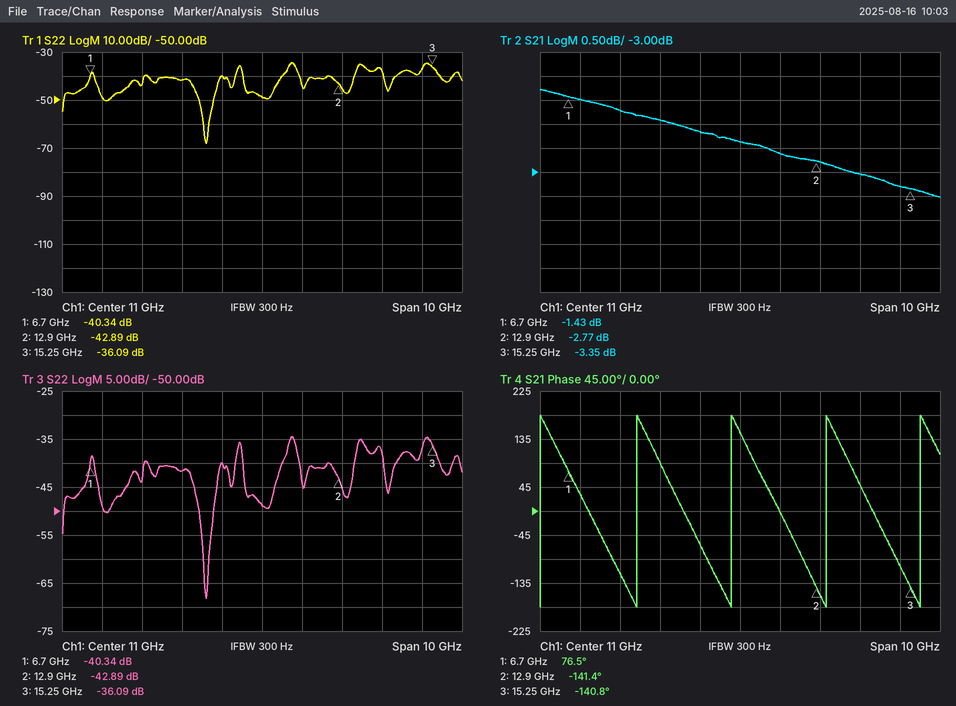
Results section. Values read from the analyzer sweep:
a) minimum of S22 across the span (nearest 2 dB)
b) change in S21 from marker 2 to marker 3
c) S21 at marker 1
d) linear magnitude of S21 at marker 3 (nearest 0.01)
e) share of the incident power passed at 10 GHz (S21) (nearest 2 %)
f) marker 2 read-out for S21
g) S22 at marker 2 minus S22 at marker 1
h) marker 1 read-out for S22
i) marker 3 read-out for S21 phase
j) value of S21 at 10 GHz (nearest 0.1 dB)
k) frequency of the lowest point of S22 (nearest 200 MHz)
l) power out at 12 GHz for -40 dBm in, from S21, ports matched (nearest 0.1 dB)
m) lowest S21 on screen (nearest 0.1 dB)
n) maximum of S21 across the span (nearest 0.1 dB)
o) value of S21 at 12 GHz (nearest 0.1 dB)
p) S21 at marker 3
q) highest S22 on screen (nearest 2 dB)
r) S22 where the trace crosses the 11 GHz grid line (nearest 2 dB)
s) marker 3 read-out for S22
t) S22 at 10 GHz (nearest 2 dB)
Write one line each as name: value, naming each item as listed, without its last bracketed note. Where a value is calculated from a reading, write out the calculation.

minimum of S22 across the span: -68 dB
change in S21 from marker 2 to marker 3: -3.35 − (-2.77) = -0.58 dB
S21 at marker 1: -1.43 dB
linear magnitude of S21 at marker 3: 10^(-3.35/20) ≈ 0.68
share of the incident power passed at 10 GHz (S21): 10^(-2.2/10) ≈ 60 %
marker 2 read-out for S21: -2.77 dB
S22 at marker 2 minus S22 at marker 1: -42.89 − (-40.34) = -2.55 dB
marker 1 read-out for S22: -40.34 dB
marker 3 read-out for S21 phase: -140.8°
value of S21 at 10 GHz: -2.2 dB
frequency of the lowest point of S22: 9.6 GHz
power out at 12 GHz for -40 dBm in, from S21, ports matched: -40 dBm + (-2.6 dB) = -42.6 dBm
lowest S21 on screen: -3.5 dB
maximum of S21 across the span: -1.3 dB
value of S21 at 12 GHz: -2.6 dB
S21 at marker 3: -3.35 dB
highest S22 on screen: -34 dB
S22 where the trace crosses the 11 GHz grid line: -48 dB
marker 3 read-out for S22: -36.09 dB
S22 at 10 GHz: -40 dB
